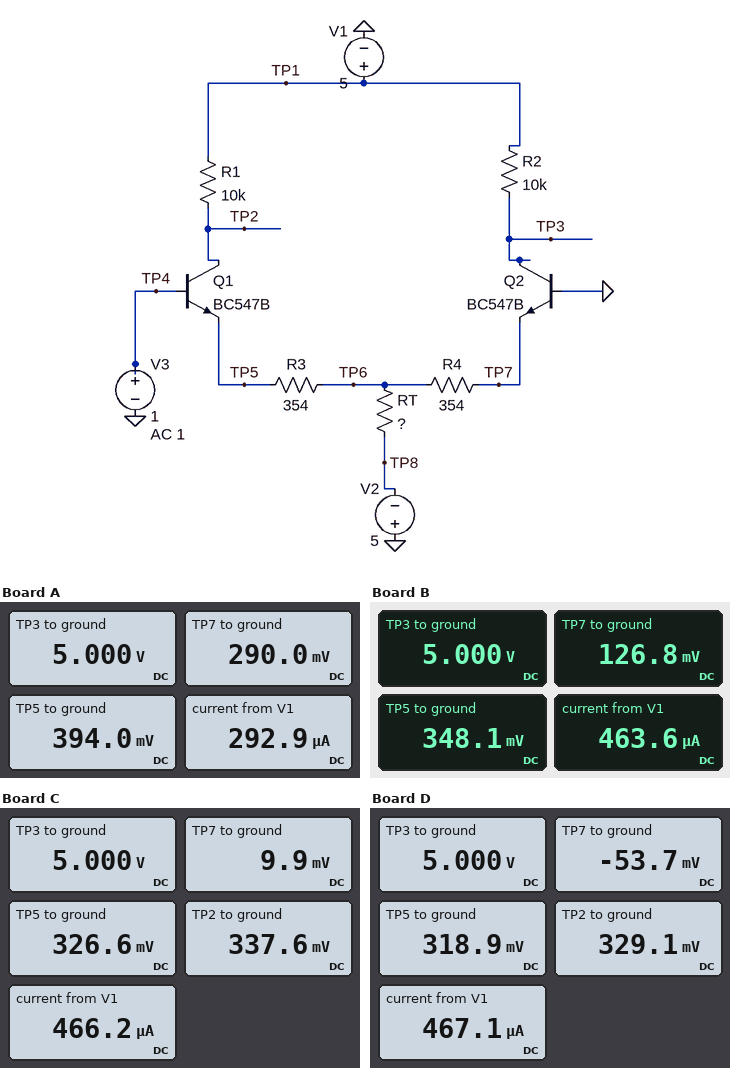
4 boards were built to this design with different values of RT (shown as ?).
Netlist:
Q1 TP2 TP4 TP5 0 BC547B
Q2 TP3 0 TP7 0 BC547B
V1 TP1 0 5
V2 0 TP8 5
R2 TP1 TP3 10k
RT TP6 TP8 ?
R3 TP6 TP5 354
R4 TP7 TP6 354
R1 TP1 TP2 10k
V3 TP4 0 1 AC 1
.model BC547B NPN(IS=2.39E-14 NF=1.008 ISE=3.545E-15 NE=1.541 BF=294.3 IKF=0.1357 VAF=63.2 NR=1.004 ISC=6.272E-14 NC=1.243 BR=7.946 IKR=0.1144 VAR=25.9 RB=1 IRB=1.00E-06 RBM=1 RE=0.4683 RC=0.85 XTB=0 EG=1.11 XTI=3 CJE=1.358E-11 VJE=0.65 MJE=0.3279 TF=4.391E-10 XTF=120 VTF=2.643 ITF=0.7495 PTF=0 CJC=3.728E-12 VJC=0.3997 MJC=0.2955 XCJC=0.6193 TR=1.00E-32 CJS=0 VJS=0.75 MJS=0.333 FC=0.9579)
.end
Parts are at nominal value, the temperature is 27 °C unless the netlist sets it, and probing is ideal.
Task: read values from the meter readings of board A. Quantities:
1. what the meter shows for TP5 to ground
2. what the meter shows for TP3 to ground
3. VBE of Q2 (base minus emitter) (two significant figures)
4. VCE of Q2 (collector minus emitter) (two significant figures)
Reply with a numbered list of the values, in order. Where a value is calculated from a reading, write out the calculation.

1. 394.0 mV
2. 5.000 V
3. 0 V - 290 mV = -290 mV
4. 5 V - 290 mV = 4.7 V
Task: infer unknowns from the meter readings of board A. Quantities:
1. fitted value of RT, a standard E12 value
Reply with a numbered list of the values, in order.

1. 18 kΩ
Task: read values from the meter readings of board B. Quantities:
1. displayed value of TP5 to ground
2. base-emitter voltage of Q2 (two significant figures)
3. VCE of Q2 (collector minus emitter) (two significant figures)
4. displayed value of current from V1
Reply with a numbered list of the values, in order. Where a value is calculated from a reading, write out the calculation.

1. 348.1 mV
2. 0 V - 126.8 mV = -130 mV
3. 5 V - 126.8 mV = 4.9 V
4. 463.6 µA
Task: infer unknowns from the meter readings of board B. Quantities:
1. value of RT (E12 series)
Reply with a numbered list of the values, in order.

1. 8.2 kΩ
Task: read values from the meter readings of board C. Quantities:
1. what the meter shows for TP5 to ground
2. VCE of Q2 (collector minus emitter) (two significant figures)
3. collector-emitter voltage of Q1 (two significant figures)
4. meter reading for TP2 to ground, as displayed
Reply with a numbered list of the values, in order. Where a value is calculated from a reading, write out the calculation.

1. 326.6 mV
2. 5 V - 9.9 mV = 5.0 V
3. 337.6 mV - 326.6 mV = 11 mV
4. 337.6 mV
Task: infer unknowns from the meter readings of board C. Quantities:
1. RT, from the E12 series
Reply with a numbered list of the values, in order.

1. 5.6 kΩ
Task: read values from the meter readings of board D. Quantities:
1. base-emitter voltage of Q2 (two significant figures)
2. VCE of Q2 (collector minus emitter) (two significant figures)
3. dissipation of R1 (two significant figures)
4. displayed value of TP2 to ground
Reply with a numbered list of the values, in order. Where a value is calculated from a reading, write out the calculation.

1. 0 V - (-53.7 mV) = 54 mV
2. 5 V - (-53.7 mV) = 5.1 V
3. (5 V - 329.1 mV)^2 / 10 kΩ = 2.2 mW
4. 329.1 mV
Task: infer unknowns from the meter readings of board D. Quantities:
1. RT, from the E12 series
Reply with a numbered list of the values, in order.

1. 4.7 kΩ
